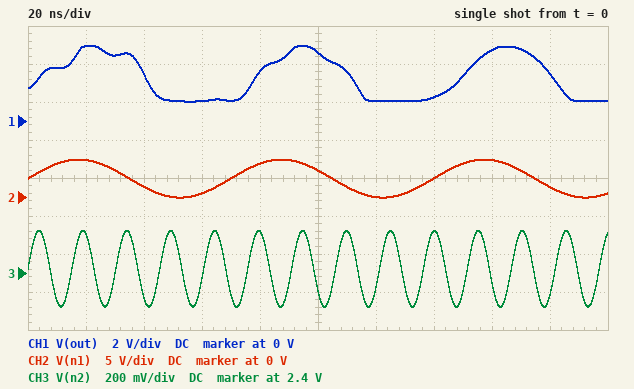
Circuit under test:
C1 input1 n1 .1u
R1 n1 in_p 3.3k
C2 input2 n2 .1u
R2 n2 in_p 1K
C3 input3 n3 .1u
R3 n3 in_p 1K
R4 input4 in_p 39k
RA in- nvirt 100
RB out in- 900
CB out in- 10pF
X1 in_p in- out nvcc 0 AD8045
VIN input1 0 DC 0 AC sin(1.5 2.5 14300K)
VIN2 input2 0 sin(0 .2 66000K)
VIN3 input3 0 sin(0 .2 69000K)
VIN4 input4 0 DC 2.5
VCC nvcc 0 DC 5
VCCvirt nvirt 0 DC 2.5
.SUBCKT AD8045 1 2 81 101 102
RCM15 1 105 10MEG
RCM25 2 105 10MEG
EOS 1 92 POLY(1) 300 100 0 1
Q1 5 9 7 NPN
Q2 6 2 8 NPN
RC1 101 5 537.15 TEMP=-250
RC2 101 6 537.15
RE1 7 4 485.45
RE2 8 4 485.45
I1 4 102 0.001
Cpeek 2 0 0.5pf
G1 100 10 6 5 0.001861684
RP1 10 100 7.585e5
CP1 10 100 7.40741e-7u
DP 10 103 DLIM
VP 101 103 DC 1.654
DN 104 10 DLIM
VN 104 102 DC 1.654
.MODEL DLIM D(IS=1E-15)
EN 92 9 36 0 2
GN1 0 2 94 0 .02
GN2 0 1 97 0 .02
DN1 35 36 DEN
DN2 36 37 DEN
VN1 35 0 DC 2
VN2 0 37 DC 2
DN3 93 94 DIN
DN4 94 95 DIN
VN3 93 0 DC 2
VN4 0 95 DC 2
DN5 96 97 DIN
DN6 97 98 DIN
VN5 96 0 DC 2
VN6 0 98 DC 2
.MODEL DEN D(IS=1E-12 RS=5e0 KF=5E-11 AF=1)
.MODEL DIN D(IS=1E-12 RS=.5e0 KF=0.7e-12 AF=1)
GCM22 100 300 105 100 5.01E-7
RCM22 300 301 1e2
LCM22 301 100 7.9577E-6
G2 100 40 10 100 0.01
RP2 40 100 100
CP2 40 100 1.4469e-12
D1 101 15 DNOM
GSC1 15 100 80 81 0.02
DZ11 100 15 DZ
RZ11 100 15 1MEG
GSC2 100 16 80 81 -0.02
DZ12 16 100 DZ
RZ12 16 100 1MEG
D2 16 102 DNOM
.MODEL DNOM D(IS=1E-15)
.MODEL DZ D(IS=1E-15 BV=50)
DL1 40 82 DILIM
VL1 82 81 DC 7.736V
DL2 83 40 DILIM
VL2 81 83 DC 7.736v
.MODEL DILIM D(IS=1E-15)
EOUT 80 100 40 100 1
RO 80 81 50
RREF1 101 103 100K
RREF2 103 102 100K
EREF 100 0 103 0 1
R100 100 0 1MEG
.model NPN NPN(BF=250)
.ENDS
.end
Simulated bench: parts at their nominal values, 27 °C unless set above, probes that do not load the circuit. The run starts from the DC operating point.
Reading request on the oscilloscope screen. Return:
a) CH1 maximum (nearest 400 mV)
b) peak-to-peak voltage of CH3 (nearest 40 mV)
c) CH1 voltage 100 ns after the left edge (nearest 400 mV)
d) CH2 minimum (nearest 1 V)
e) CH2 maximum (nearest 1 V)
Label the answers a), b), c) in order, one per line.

a) 4.0 V
b) 400 mV
c) 3.6 V
d) 0 V
e) 5 V
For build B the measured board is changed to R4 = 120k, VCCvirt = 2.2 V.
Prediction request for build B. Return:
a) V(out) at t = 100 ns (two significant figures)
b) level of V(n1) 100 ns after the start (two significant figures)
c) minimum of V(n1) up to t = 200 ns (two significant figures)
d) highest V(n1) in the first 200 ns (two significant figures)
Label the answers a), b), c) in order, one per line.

a) 3.8 V
b) 3.3 V
c) -240 mV
d) 4.8 V
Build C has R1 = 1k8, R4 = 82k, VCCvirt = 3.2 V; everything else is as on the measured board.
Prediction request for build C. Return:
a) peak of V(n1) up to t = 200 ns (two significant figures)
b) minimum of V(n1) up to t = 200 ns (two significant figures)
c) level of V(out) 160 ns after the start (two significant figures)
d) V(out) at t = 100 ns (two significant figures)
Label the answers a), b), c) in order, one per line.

a) 5.0 V
b) -17 mV
c) 1.2 V
d) 1.1 V
